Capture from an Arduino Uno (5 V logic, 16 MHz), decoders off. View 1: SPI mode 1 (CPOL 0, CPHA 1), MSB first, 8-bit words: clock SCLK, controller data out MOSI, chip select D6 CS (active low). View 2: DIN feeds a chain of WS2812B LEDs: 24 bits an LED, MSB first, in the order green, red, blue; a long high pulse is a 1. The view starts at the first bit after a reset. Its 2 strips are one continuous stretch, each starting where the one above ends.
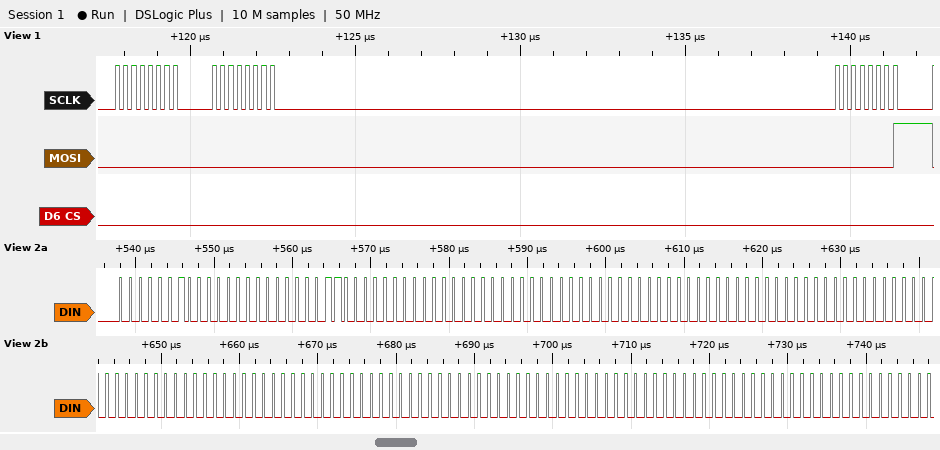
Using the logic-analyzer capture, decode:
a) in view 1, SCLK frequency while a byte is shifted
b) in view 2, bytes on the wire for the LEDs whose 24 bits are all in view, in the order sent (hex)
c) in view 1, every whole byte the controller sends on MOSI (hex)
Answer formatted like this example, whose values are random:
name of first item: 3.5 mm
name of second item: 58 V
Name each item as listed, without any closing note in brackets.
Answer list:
in view 1, SCLK frequency while a byte is shifted: 4 MHz
in view 2, bytes on the wire for the LEDs whose 24 bits are all in view, in the order sent: 02 00 06 00 00 00 00 00 00 00 00 00 00 00 00 00 00 00 00 00 00
in view 1, every whole byte the controller sends on MOSI: 00 00 01
